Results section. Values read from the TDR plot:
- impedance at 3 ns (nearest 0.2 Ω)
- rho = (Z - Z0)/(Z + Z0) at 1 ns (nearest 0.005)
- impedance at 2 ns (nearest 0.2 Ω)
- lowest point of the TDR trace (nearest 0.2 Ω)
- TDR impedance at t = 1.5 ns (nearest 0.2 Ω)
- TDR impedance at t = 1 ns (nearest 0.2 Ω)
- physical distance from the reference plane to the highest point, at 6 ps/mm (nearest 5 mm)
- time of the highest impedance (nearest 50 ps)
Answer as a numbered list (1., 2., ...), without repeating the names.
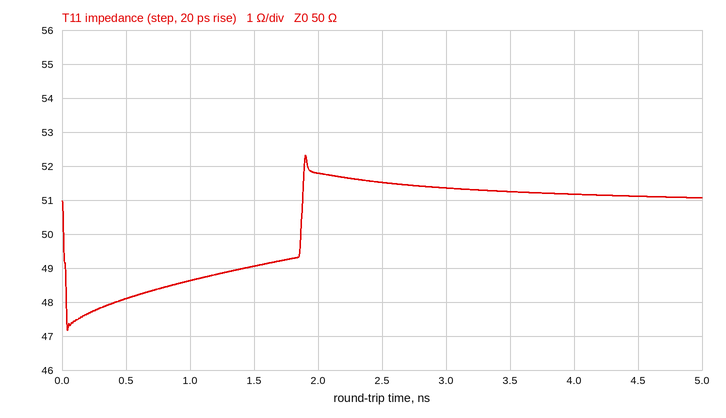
1. 51.4 Ω
2. -0.015
3. 51.8 Ω
4. 47.2 Ω
5. 49.0 Ω
6. 48.6 Ω
7. 160 mm
8. 1.90 ns
